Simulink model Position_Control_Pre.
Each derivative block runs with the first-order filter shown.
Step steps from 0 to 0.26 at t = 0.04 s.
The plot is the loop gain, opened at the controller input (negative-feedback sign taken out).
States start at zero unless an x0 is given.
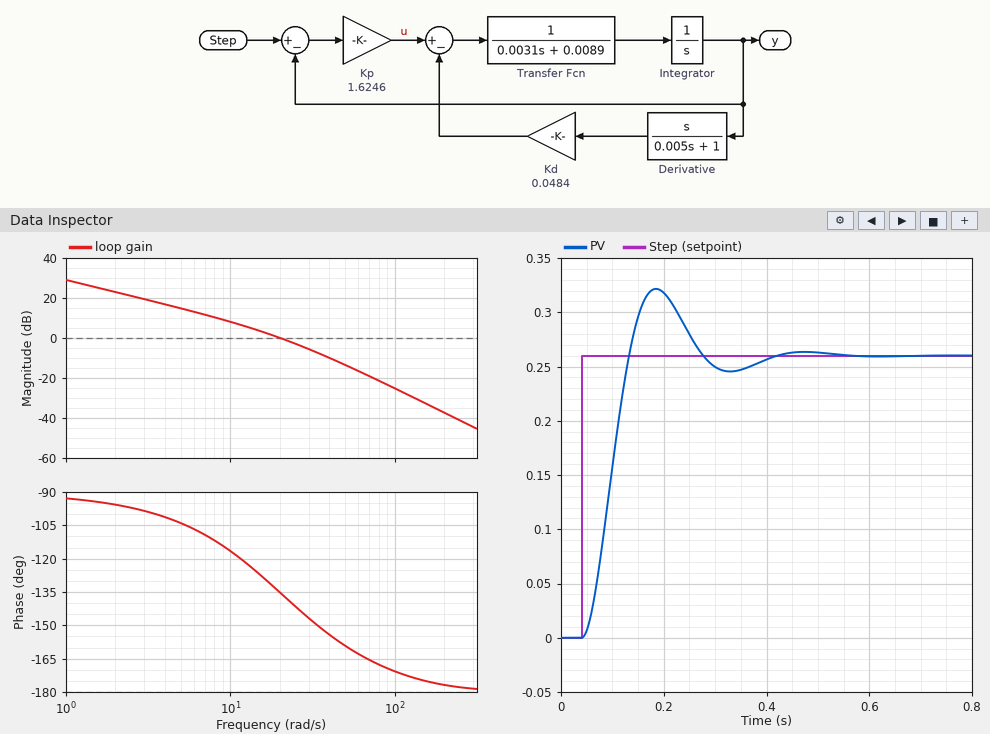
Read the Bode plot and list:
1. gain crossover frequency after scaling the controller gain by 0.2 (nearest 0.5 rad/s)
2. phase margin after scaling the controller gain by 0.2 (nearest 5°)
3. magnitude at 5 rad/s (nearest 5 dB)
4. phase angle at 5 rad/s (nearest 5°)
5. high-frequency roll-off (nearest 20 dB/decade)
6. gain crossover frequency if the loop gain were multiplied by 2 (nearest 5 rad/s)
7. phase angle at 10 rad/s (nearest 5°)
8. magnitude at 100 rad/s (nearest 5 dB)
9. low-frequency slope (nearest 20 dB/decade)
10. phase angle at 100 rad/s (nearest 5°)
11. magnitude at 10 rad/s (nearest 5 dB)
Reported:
5.5 rad/s
75°
15 dB
-105°
-40 dB/decade
30 rad/s
-115°
-25 dB
-20 dB/decade
-170°
10 dB
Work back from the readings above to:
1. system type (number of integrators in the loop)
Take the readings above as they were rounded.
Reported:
1
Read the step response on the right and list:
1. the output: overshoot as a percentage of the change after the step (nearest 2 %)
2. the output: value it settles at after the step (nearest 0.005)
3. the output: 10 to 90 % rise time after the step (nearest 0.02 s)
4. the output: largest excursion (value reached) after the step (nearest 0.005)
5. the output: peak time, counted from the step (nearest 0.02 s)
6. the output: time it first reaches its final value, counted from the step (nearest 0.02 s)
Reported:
24 %
0.260
0.06 s
0.320
0.14 s
0.10 s
